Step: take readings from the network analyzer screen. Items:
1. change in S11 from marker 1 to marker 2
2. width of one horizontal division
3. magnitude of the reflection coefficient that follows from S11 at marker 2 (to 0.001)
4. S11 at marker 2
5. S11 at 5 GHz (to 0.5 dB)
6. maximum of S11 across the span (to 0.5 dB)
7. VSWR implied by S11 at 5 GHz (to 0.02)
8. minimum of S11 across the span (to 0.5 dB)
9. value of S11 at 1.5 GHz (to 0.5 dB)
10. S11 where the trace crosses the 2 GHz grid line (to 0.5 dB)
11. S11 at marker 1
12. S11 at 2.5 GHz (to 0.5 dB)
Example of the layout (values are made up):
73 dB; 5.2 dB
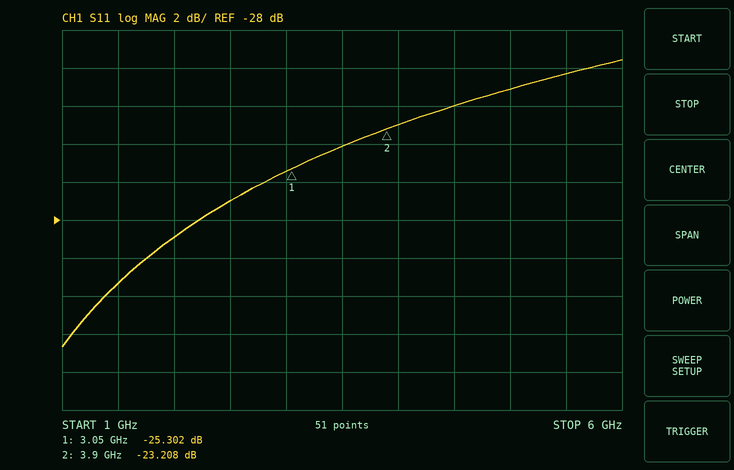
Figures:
2.094 dB; 500 MHz; 0.069; -23.208 dB; -21.0 dB; -19.5 dB; 1.20; -34.5 dB; -31.5 dB; -29.0 dB; -25.302 dB; -27.0 dB
